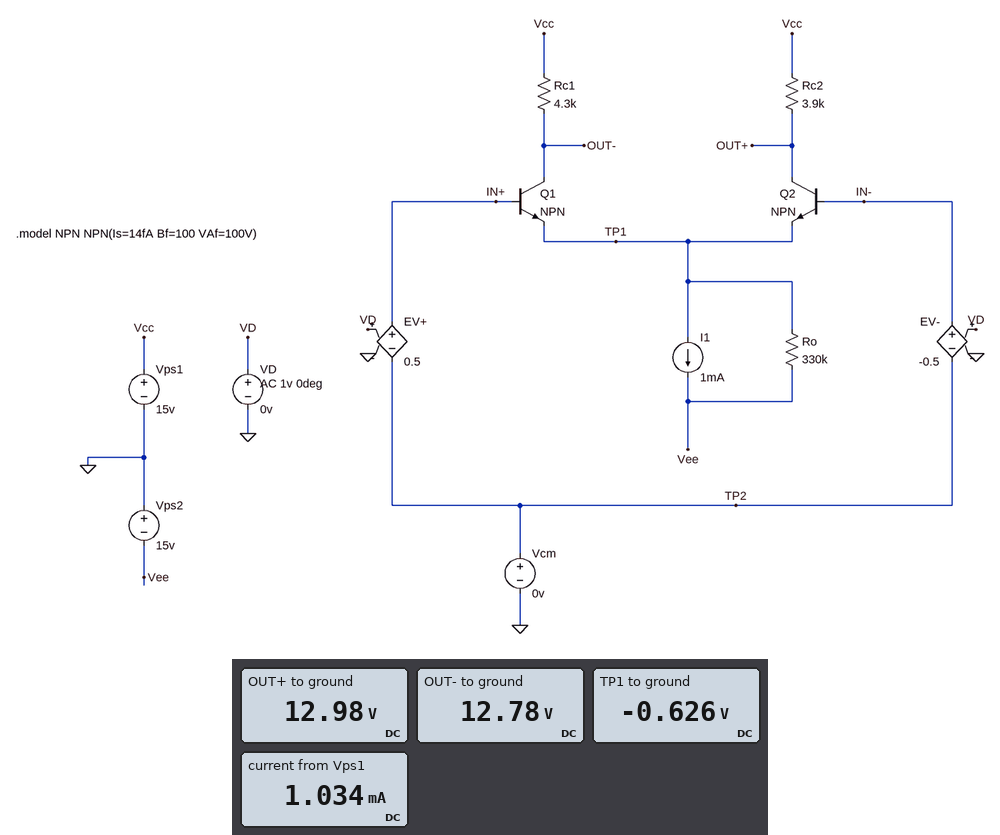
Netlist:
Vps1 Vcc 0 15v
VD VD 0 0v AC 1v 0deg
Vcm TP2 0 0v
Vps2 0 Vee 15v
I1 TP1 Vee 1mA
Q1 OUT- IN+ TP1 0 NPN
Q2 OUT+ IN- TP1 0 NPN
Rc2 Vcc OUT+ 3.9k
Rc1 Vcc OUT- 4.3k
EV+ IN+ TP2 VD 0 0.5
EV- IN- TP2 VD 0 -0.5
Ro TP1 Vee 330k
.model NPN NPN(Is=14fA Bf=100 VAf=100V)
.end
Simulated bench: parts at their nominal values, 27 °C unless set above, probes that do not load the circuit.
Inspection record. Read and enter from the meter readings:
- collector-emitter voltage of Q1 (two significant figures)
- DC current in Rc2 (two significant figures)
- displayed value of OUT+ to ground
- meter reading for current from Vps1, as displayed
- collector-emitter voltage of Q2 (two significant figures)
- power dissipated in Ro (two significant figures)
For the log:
13 V
520 µA
12.98 V
1.034 mA
14 V
630 µW
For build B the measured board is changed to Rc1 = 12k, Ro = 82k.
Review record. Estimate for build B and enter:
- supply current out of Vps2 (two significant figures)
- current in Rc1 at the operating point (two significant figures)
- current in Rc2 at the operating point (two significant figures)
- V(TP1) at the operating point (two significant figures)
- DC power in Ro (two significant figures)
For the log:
1.2 mA
570 µA
590 µA
-630 mV
2.5 mW
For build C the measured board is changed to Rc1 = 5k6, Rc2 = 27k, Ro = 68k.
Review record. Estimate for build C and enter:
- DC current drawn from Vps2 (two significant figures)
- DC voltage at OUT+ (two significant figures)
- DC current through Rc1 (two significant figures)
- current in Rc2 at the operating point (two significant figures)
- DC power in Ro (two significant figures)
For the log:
1.2 mA
-300 mV
630 µA
570 µA
3.0 mW
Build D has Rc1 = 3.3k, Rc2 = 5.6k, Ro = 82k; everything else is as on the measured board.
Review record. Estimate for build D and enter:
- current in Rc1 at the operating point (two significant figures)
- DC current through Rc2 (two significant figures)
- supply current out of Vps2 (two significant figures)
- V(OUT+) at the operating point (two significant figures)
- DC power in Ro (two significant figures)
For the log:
590 µA
580 µA
1.2 mA
12 V
2.5 mW
